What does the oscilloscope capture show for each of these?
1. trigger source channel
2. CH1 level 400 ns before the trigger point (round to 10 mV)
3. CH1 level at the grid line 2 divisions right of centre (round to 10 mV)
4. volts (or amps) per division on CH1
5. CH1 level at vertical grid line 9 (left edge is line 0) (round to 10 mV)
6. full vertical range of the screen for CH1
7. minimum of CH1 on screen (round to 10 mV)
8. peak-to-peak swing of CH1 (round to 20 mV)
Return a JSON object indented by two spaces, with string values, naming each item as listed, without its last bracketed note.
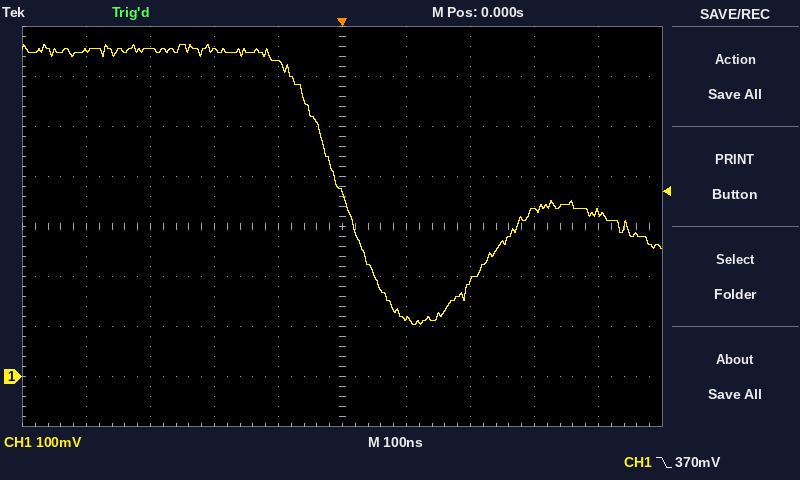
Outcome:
{
  "trigger source channel": "CH1",
  "CH1 level 400 ns before the trigger point": "650 mV",
  "CH1 level at the grid line 2 divisions right of centre": "190 mV",
  "volts (or amps) per division on CH1": "100 mV",
  "CH1 level at vertical grid line 9 (left edge is line 0)": "330 mV",
  "full vertical range of the screen for CH1": "800 mV",
  "minimum of CH1 on screen": "100 mV",
  "peak-to-peak swing of CH1": "560 mV"
}
